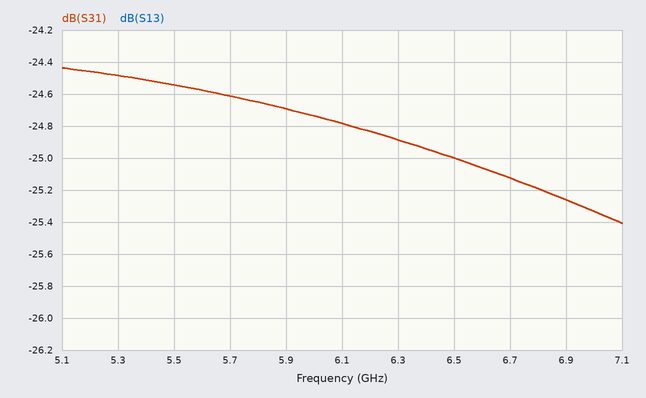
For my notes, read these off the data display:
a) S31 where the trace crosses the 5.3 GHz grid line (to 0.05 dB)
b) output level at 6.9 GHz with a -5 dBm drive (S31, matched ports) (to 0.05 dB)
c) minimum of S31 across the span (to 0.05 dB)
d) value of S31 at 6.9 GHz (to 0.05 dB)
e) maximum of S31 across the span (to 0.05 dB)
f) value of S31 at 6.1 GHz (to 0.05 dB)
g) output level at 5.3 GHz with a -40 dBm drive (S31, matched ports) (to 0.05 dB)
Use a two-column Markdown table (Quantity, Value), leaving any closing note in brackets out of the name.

| Quantity | Value |
|---|---|
| S31 where the trace crosses the 5.3 GHz grid line | -24.50 dB |
| output level at 6.9 GHz with a -5 dBm drive (S31, matched ports) | -30.25 dBm |
| minimum of S31 across the span | -25.40 dB |
| value of S31 at 6.9 GHz | -25.25 dB |
| maximum of S31 across the span | -24.45 dB |
| value of S31 at 6.1 GHz | -24.80 dB |
| output level at 5.3 GHz with a -40 dBm drive (S31, matched ports) | -64.50 dBm |
